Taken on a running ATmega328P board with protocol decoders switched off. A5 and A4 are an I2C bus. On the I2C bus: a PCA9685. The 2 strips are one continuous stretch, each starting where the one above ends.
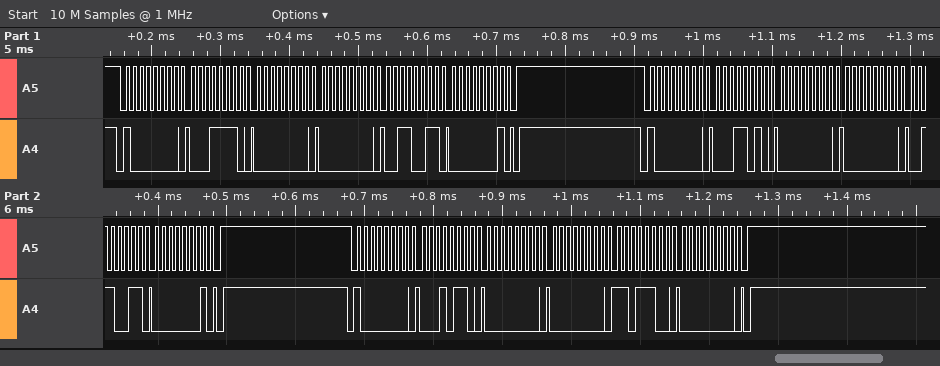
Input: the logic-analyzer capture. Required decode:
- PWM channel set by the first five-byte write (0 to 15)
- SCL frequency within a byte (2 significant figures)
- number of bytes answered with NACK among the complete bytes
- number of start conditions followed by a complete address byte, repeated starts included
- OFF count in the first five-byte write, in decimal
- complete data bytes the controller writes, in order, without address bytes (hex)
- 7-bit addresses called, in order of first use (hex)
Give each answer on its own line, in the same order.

6
100 kHz
0
3
307
1E 00 00 33 01 1A 00 00 33 01 16 00 00 DC 00
0x40
